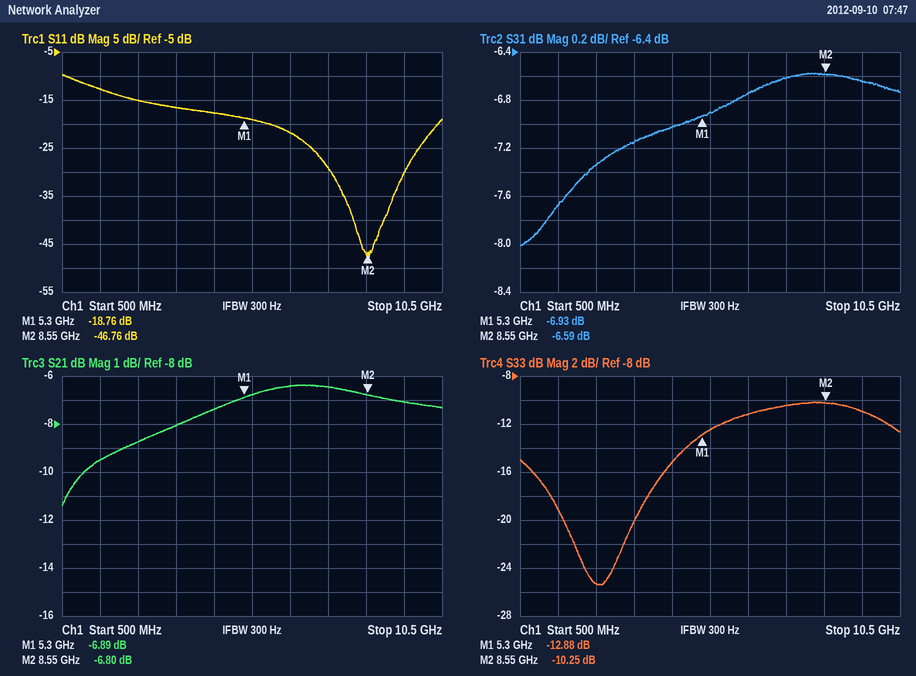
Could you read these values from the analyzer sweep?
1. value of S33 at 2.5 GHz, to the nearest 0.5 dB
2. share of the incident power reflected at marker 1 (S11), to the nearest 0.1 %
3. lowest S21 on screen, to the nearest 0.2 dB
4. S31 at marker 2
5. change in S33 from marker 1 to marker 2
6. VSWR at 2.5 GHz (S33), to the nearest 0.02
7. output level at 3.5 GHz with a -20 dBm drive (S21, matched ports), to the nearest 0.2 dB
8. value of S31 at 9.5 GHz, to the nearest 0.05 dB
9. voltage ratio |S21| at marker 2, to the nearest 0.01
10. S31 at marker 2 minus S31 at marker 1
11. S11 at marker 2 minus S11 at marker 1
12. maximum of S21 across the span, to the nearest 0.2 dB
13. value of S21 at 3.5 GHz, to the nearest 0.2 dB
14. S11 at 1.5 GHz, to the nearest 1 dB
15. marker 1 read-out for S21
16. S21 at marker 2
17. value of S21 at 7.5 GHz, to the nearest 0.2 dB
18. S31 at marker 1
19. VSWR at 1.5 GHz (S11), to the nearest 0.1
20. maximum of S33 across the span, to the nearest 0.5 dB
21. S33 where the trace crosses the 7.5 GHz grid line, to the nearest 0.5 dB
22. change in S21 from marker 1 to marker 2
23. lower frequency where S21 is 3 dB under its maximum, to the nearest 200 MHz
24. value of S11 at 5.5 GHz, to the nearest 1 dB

-25.5 dB
1.3 %
-11.4 dB
-6.59 dB
2.63 dB
1.12
-28.0 dBm
-6.65 dB
0.46
0.34 dB
-28.00 dB
-6.4 dB
-8.0 dB
-13 dB
-6.89 dB
-6.80 dB
-6.4 dB
-6.93 dB
1.6
-10.0 dB
-10.5 dB
0.09 dB
1.6 GHz
-19 dB
